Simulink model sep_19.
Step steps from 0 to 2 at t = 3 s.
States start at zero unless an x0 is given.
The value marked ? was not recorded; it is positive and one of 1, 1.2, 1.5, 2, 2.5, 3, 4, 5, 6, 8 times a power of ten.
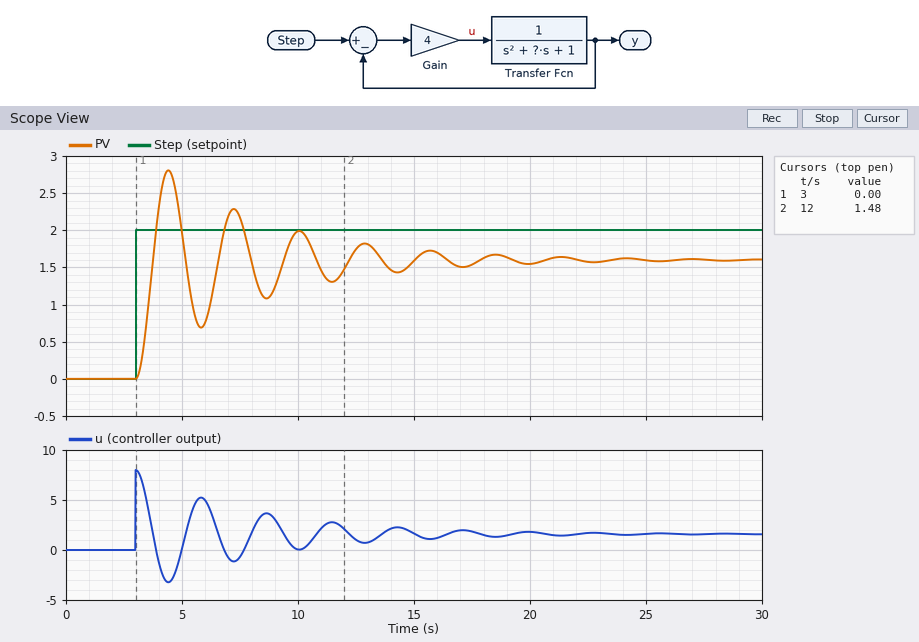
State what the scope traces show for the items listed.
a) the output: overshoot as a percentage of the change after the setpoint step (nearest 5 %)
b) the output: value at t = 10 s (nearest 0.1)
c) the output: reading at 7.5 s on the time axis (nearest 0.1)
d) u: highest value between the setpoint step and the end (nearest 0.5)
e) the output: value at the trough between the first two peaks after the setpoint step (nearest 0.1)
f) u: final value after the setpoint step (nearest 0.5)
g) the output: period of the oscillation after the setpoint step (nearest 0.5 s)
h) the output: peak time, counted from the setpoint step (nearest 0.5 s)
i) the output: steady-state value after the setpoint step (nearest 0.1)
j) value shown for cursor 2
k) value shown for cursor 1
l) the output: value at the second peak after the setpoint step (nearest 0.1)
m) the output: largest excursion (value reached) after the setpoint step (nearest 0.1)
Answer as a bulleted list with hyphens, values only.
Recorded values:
- 75 %
- 2.0
- 2.2
- 8.0
- 0.7
- 1.5
- 3.0 s
- 1.5 s
- 1.6
- 1.48
- 0.00
- 2.3
- 2.8
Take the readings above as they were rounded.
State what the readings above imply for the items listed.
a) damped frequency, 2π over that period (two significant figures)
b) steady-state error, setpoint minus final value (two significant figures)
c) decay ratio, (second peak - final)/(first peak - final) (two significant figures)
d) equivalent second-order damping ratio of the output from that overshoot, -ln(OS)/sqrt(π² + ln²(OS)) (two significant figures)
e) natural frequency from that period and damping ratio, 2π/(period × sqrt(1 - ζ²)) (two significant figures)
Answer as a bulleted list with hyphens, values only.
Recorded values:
- 2.1 rad/s
- 0.40
- 0.58
- 0.091
- 2.1 rad/s
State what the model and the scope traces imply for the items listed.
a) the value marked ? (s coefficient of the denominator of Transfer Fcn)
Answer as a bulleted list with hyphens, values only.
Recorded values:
- 0.4
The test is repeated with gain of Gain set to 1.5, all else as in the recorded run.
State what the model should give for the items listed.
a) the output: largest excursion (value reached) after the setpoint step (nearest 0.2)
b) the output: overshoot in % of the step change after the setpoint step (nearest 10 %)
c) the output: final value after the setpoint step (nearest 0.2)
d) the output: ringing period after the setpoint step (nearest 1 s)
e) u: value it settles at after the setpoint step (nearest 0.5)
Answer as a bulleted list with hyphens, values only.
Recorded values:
- 2.0
- 70 %
- 1.2
- 4 s
- 1.0
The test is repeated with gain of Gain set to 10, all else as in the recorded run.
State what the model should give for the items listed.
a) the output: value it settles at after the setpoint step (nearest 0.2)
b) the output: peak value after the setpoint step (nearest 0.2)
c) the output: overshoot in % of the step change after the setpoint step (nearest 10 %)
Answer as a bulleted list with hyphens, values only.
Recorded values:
- 1.8
- 3.4
- 80 %
